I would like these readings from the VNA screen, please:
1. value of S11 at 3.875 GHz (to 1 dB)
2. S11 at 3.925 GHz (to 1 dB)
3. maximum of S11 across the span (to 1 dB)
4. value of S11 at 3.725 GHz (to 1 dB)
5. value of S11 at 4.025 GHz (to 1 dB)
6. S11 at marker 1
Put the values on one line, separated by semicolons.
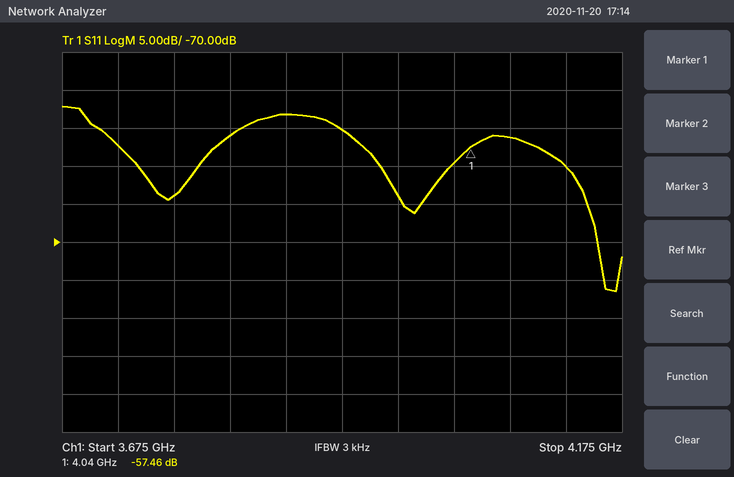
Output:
-53 dB; -55 dB; -52 dB; -57 dB; -60 dB; -57.46 dB
